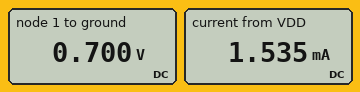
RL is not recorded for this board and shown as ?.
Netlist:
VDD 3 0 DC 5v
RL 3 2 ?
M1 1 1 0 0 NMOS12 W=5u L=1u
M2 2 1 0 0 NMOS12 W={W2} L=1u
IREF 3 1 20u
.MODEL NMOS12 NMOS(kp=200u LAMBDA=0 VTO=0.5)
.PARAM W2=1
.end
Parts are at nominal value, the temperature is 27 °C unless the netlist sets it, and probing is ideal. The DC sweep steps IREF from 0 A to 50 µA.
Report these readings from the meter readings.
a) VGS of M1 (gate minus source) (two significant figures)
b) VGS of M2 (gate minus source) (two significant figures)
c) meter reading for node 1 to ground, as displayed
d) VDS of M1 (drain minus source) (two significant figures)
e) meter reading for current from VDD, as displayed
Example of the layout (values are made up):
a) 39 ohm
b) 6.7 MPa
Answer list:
a) 700 mV
b) 700 mV
c) 0.700 V
d) 700 mV
e) 1.535 mA
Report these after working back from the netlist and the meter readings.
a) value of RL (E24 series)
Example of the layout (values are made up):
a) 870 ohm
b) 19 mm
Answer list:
a) 3.3 kΩ
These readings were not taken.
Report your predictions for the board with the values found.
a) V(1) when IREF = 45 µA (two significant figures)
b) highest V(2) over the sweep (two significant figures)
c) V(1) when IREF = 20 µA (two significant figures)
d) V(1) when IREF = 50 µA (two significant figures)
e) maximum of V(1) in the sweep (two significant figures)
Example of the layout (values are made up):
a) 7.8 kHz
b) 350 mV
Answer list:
a) 800 mV
b) 5.0 V
c) 700 mV
d) 820 mV
e) 820 mV
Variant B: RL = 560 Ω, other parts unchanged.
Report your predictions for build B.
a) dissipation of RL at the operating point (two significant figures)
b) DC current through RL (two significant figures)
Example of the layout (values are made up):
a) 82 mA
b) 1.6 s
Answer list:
a) 45 mW
b) 8.9 mA
